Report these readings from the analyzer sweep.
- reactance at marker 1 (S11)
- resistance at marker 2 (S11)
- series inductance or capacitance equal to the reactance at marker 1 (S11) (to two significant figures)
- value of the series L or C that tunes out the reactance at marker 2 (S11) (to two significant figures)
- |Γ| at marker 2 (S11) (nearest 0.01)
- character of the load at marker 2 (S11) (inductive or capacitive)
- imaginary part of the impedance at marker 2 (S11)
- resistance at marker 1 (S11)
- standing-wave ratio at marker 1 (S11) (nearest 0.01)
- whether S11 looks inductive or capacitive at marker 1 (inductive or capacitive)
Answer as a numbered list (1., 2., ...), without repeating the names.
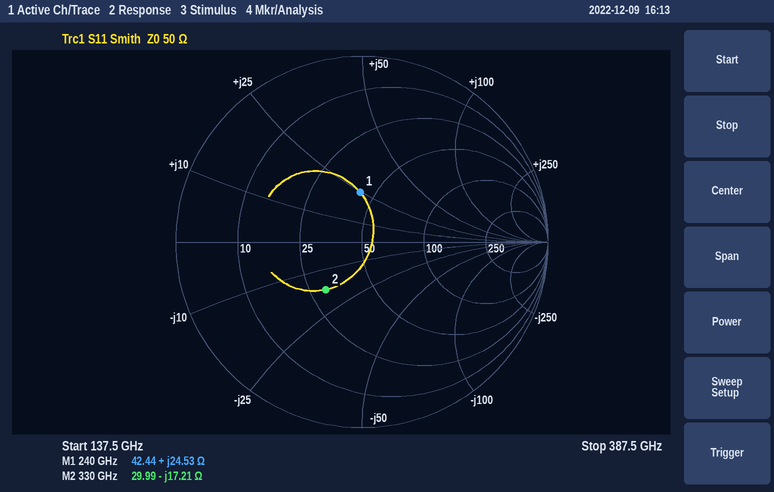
1. +24.53 Ω
2. 29.99 Ω
3. 16 pH
4. 8.3 pH
5. 0.32
6. capacitive
7. -17.21 Ω
8. 42.44 Ω
9. 1.73
10. inductive
